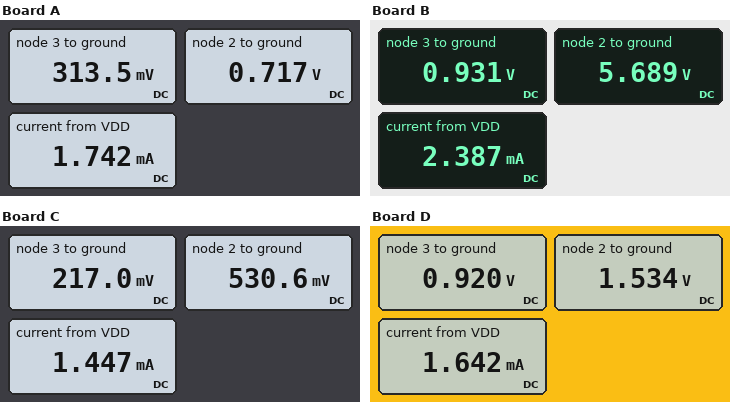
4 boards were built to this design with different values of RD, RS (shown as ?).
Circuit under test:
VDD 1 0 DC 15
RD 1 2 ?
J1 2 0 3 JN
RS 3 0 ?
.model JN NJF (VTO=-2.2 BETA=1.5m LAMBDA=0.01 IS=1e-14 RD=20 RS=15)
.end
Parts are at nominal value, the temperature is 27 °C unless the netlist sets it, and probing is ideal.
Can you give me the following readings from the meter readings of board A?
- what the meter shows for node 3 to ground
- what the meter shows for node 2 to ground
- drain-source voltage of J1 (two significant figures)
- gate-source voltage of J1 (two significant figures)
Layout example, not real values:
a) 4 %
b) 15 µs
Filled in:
a) 313.5 mV
b) 0.717 V
c) 400 mV
d) -310 mV
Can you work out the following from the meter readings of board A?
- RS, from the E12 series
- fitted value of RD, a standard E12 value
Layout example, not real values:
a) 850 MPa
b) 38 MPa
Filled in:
a) 180 Ω
b) 8.2 kΩ
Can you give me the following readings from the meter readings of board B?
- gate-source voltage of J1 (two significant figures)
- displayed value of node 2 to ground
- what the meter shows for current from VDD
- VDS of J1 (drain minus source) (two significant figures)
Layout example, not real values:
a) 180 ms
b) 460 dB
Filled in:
a) -930 mV
b) 5.689 V
c) 2.387 mA
d) 4.8 V
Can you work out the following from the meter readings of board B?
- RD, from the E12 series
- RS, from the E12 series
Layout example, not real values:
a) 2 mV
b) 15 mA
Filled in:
a) 3.9 kΩ
b) 390 Ω
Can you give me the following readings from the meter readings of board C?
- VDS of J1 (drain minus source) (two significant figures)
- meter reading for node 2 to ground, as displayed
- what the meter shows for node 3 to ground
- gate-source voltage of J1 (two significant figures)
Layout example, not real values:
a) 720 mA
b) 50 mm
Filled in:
a) 310 mV
b) 530.6 mV
c) 217.0 mV
d) -220 mV
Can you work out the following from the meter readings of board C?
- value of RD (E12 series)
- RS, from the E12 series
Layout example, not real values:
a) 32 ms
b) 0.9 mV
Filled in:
a) 10 kΩ
b) 150 Ω
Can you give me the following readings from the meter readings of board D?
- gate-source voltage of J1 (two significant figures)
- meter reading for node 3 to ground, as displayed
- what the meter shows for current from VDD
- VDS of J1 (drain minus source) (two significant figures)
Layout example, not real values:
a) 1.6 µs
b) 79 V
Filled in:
a) -920 mV
b) 0.920 V
c) 1.642 mA
d) 610 mV
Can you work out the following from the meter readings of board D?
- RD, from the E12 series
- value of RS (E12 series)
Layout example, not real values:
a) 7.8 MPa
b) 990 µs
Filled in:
a) 8.2 kΩ
b) 560 Ω
